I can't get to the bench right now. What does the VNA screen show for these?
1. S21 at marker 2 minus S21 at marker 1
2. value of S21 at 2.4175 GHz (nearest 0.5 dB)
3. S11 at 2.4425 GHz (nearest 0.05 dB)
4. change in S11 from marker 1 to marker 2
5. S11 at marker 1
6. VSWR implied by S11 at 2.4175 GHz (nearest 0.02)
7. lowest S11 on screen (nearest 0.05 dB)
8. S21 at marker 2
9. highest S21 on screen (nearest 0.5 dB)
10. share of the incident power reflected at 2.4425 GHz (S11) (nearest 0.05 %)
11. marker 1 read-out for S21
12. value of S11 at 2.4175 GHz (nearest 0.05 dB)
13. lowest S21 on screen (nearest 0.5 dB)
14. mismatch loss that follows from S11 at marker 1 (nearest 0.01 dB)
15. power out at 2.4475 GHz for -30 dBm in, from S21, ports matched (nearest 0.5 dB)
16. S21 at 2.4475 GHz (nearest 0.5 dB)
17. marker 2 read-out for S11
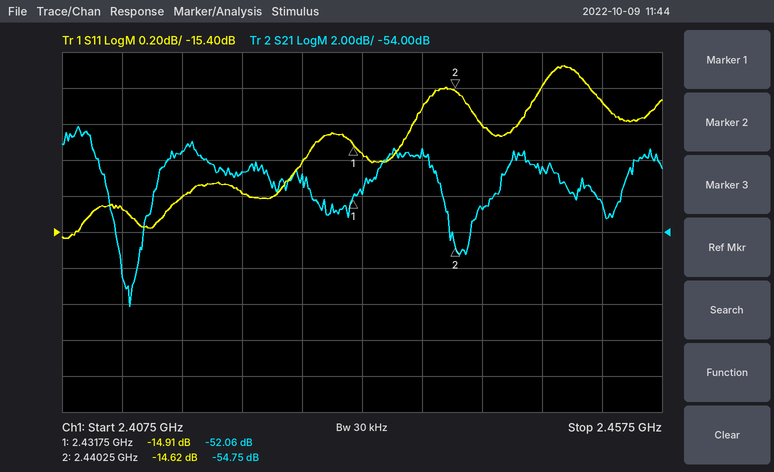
-2.69 dB
-49.5 dB
-14.80 dB
0.29 dB
-14.91 dB
1.42
-15.45 dB
-54.75 dB
-48.0 dB
3.30 %
-52.06 dB
-15.20 dB
-58.0 dB
0.14 dB
-80.5 dBm
-50.5 dB
-14.62 dB
